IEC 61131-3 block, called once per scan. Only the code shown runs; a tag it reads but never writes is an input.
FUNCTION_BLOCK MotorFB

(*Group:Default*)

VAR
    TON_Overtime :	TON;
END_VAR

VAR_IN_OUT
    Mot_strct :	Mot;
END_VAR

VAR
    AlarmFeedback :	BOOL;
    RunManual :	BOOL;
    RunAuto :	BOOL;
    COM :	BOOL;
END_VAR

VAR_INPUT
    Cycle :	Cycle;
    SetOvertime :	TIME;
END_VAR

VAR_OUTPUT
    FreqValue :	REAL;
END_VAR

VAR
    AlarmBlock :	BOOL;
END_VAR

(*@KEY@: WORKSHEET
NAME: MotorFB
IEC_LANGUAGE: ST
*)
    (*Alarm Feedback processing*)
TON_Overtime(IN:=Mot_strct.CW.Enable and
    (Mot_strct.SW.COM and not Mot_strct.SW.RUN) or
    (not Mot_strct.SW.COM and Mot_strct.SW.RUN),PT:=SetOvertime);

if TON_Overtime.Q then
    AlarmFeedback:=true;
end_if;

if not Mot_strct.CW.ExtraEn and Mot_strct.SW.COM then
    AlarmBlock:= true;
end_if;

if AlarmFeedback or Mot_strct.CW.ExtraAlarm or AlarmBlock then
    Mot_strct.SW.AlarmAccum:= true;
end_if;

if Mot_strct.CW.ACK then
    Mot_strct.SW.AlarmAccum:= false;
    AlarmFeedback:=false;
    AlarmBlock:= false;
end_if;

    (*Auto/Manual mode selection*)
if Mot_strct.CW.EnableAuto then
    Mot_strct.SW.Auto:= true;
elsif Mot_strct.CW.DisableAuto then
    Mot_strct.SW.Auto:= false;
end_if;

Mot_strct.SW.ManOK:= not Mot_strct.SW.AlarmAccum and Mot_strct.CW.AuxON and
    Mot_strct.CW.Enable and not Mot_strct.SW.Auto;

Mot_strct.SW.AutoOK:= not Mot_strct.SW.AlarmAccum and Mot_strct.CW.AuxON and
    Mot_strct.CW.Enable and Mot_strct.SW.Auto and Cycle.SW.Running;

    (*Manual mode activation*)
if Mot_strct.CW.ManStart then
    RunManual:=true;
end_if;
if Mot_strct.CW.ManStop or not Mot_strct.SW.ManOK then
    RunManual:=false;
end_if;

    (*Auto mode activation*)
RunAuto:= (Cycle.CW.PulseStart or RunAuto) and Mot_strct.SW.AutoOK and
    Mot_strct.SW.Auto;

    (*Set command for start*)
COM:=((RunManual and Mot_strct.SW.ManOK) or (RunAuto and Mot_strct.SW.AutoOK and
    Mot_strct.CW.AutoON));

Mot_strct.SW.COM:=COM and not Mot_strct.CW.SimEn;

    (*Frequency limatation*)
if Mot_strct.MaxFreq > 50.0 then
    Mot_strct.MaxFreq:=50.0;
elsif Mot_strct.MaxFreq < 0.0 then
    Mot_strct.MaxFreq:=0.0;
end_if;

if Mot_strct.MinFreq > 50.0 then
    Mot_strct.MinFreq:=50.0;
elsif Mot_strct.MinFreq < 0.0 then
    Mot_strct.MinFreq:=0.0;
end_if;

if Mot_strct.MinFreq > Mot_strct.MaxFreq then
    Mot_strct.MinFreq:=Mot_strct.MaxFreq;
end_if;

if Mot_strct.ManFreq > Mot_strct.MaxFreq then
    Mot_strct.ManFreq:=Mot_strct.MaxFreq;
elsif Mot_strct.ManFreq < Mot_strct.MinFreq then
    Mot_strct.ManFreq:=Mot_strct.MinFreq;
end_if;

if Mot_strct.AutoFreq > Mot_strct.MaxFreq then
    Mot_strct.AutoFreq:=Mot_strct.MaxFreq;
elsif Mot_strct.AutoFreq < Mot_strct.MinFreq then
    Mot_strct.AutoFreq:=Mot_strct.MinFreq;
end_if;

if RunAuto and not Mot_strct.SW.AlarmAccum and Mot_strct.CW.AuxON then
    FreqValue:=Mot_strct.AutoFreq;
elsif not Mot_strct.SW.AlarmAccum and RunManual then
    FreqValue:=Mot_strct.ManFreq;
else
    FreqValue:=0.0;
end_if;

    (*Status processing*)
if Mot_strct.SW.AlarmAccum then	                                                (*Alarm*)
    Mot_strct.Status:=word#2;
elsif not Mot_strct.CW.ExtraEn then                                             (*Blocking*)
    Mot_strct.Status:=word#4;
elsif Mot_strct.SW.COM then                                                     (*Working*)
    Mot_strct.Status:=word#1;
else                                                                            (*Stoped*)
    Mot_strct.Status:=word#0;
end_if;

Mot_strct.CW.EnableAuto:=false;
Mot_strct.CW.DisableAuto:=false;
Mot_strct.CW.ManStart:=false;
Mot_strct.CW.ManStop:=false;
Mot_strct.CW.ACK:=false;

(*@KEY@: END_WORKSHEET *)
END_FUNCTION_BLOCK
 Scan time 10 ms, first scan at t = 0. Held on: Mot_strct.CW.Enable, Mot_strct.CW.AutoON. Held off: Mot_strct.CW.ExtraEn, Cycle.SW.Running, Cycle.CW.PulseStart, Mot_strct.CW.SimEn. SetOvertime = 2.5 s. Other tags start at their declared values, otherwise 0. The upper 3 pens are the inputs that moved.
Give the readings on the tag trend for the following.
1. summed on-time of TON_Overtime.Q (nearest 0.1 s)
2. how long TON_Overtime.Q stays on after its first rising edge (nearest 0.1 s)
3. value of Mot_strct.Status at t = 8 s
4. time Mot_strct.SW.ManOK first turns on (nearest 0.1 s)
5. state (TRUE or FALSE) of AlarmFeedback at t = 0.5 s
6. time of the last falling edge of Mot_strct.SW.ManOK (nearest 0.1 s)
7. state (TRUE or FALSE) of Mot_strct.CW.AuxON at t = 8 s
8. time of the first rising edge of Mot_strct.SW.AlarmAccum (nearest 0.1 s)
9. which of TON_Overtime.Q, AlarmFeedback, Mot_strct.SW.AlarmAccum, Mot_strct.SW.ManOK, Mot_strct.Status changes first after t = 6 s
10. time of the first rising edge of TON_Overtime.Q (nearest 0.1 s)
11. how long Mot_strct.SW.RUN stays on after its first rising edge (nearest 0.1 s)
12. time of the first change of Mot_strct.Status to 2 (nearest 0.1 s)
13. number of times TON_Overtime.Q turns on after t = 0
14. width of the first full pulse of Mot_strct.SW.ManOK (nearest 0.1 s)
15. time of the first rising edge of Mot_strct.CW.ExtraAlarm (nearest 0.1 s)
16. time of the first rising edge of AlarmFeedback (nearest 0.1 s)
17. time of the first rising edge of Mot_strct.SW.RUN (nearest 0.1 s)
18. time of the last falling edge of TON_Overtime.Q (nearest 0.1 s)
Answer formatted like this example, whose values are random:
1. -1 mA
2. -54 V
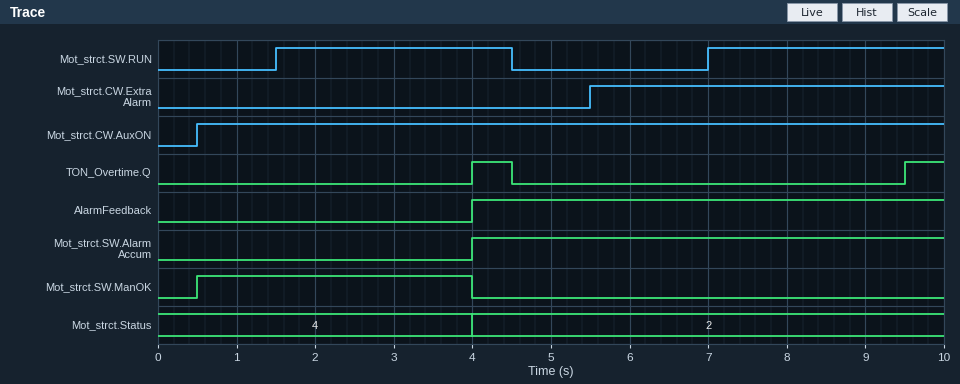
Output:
1. 1.0 s
2. 0.5 s
3. 2
4. 0.5 s
5. FALSE
6. 4.0 s
7. TRUE
8. 4.0 s
9. TON_Overtime.Q
10. 4.0 s
11. 3.0 s
12. 4.0 s
13. 2
14. 3.5 s
15. 5.5 s
16. 4.0 s
17. 1.5 s
18. 4.5 s
